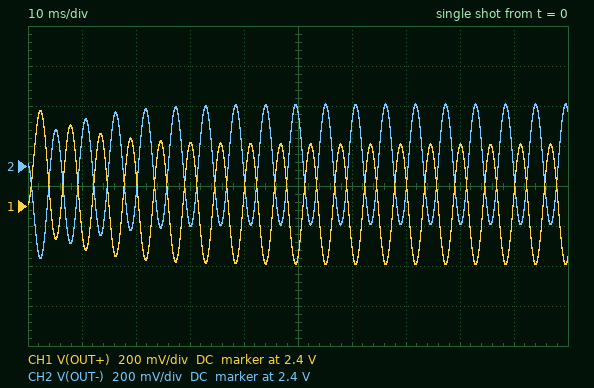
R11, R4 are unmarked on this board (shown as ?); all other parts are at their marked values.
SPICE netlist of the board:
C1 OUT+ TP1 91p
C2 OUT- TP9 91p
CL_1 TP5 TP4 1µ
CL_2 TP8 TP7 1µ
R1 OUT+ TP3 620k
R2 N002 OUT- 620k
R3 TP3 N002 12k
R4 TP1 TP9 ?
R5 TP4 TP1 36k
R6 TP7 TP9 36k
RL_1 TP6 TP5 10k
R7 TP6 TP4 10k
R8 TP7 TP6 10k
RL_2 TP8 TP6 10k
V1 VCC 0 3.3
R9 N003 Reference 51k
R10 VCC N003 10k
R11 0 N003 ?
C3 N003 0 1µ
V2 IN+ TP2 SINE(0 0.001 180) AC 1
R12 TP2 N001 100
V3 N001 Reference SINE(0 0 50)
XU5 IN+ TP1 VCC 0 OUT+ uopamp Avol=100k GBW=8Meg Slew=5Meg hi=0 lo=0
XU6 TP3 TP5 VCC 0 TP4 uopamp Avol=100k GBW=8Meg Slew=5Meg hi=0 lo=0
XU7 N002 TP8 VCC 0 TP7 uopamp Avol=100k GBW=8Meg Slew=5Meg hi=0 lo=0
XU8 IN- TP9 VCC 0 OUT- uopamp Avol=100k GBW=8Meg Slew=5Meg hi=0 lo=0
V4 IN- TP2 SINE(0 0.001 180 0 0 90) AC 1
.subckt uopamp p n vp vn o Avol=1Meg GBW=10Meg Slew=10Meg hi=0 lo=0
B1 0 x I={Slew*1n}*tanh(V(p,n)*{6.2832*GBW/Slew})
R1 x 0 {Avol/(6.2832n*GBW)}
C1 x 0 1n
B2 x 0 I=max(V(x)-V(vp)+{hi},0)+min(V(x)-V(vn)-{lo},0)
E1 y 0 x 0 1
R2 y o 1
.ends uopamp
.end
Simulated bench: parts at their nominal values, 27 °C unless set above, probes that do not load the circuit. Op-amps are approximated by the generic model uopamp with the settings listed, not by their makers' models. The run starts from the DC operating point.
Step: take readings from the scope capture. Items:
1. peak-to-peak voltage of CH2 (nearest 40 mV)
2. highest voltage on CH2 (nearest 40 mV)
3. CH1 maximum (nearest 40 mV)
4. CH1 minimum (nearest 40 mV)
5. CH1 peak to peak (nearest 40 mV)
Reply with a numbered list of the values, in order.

1. 760 mV
2. 2.72 V
3. 2.88 V
4. 2.12 V
5. 760 mV
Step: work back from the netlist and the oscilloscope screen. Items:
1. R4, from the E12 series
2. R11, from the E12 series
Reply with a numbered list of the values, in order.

1. 22 kΩ
2. 27 kΩ
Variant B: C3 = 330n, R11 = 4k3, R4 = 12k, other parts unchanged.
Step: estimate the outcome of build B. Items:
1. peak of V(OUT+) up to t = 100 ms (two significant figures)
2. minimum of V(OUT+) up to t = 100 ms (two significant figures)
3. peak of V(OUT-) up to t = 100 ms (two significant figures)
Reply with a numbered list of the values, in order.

1. 1.8 V
2. 500 mV
3. 1.5 V
